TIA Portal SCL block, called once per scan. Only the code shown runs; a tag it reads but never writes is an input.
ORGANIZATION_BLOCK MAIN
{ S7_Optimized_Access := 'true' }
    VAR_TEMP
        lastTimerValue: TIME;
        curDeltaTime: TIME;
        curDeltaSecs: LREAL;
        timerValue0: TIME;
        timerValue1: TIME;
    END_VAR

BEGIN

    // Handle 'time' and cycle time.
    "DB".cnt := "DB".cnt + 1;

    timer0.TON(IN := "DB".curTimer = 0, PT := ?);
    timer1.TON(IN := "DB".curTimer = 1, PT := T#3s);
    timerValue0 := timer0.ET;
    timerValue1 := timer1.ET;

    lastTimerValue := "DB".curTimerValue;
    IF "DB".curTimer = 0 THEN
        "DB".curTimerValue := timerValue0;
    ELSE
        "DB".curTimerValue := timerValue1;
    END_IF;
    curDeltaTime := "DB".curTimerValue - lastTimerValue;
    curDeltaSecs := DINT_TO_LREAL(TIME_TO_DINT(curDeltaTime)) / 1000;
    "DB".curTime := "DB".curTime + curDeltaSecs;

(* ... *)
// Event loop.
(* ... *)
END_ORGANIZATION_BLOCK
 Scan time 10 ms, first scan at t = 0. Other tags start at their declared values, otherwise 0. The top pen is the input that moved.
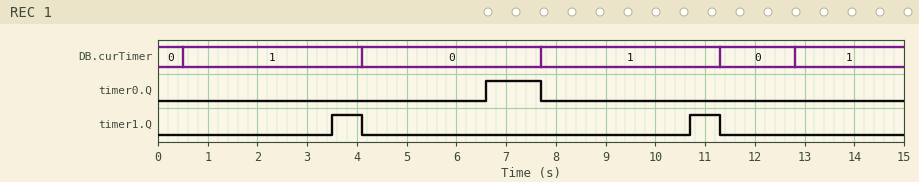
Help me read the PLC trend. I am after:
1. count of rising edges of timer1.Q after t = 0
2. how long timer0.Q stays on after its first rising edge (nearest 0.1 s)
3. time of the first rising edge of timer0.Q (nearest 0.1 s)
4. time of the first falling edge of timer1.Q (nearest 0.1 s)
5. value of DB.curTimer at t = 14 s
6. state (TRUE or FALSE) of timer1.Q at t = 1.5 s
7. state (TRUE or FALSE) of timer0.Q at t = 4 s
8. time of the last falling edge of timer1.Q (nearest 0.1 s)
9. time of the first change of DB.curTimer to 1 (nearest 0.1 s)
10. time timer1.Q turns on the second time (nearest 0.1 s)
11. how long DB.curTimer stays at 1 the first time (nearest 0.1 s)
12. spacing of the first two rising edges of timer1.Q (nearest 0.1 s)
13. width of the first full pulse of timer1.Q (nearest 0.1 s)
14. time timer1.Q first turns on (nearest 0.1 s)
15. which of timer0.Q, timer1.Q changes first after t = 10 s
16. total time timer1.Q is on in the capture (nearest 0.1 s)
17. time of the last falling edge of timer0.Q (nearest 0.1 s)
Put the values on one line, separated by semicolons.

2; 1.1 s; 6.6 s; 4.1 s; 1; FALSE; FALSE; 11.3 s; 0.5 s; 10.7 s; 3.6 s; 7.2 s; 0.6 s; 3.5 s; timer1.Q; 1.2 s; 7.7 s
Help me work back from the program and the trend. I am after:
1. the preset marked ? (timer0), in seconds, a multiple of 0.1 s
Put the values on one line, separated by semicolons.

2.5 s
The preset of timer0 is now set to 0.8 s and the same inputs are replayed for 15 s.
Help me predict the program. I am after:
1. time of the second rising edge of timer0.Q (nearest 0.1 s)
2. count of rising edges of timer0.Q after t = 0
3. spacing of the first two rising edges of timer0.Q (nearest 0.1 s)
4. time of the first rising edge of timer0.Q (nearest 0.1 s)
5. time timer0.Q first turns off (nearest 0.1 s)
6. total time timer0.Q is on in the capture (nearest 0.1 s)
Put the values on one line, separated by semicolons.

12.1 s; 2; 7.2 s; 4.9 s; 7.7 s; 3.5 s
